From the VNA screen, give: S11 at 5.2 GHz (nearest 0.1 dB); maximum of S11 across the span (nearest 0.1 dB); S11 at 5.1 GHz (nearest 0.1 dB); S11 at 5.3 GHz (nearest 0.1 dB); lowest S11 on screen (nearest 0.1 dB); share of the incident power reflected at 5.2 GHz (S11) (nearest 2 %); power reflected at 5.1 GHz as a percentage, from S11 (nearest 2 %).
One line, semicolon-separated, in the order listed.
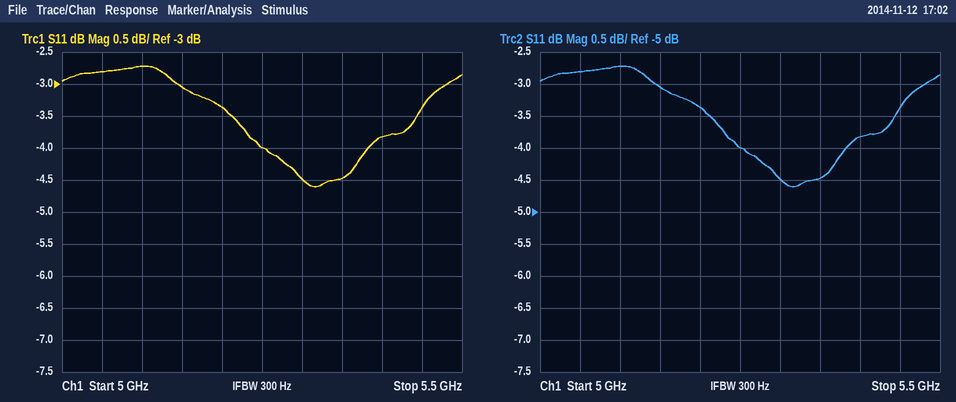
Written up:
-3.4 dB; -2.7 dB; -2.7 dB; -4.5 dB; -4.6 dB; 46 %; 54 %
